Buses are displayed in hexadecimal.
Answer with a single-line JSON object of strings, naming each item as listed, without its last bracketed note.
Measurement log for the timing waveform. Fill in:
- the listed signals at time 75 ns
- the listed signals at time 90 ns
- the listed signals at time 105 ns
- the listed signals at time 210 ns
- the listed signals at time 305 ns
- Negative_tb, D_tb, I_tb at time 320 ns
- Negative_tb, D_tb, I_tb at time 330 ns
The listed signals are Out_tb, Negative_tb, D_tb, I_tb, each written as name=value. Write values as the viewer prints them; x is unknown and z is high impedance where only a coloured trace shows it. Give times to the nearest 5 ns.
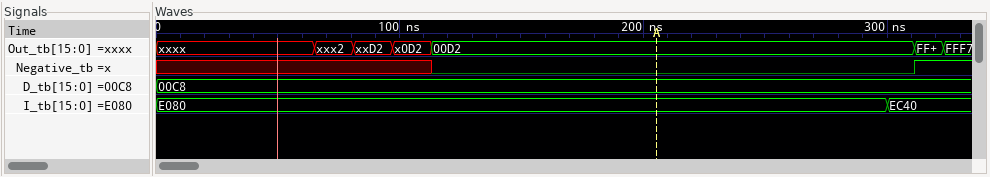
{"the listed signals at time 75 ns": "Out_tb=xxx2, Negative_tb=x, D_tb=00C8, I_tb=E080", "the listed signals at time 90 ns": "Out_tb=xxD2, Negative_tb=x, D_tb=00C8, I_tb=E080", "the listed signals at time 105 ns": "Out_tb=x0D2, Negative_tb=x, D_tb=00C8, I_tb=E080", "the listed signals at time 210 ns": "Out_tb=00D2, Negative_tb=0, D_tb=00C8, I_tb=E080", "the listed signals at time 305 ns": "Out_tb=00D2, Negative_tb=0, D_tb=00C8, I_tb=EC40", "Negative_tb, D_tb, I_tb at time 320 ns": "Negative_tb=1, D_tb=00C8, I_tb=EC40", "Negative_tb, D_tb, I_tb at time 330 ns": "Negative_tb=1, D_tb=00C8, I_tb=EC40"}
